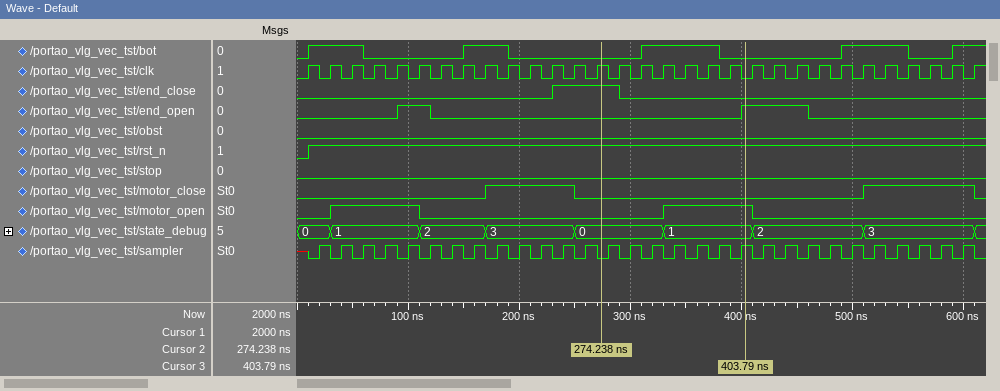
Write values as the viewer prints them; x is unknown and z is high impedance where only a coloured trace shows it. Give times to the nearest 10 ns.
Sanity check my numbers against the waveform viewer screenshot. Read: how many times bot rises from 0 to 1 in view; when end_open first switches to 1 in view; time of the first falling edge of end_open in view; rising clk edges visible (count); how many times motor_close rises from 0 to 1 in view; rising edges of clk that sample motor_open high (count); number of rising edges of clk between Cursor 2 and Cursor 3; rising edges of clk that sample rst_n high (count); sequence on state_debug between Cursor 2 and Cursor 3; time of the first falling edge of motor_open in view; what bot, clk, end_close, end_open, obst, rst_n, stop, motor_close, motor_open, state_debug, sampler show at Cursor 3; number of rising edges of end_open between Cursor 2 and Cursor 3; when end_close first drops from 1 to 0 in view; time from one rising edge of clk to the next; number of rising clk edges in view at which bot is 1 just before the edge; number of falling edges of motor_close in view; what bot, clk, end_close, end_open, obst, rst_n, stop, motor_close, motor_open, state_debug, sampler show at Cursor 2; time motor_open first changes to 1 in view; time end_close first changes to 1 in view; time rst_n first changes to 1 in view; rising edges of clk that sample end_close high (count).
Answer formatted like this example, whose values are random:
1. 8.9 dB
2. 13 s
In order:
1. 5
2. 90 ns
3. 120 ns
4. 31
5. 2
6. 8
7. 6
8. 30
9. 0, 1
10. 110 ns
11. bot=0, clk=0, end_close=0, end_open=1, obst=0, rst_n=1, stop=0, motor_close=0, motor_open=1, state_debug=1, sampler=1
12. 1
13. 290 ns
14. 20 ns
15. 11
16. 2
17. bot=0, clk=1, end_close=1, end_open=0, obst=0, rst_n=1, stop=0, motor_close=0, motor_open=0, state_debug=0, sampler=0
18. 30 ns
19. 230 ns
20. 10 ns
21. 3
